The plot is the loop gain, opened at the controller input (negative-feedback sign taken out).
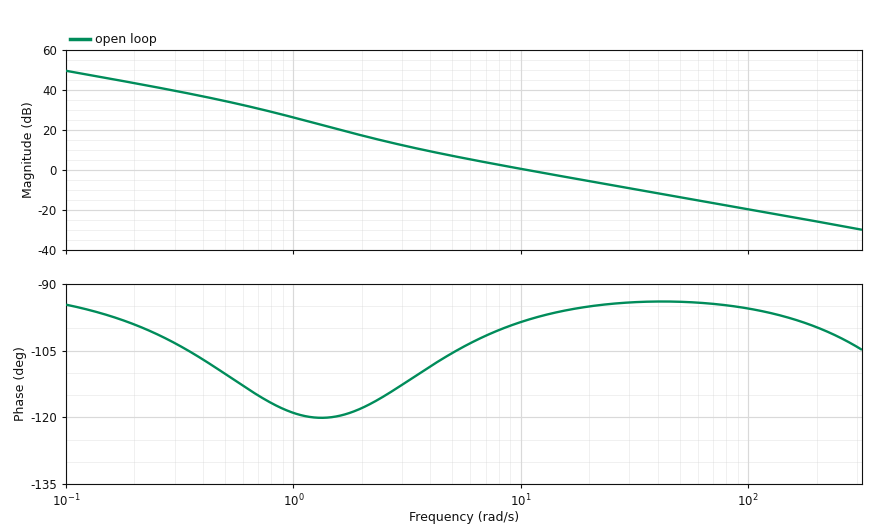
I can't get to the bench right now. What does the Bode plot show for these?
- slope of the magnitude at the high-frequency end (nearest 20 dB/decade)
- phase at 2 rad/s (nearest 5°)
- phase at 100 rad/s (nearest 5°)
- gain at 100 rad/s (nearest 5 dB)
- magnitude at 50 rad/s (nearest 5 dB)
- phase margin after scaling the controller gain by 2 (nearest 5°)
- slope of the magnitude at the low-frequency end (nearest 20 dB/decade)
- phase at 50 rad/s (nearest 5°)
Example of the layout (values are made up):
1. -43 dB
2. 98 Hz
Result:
1. -20 dB/decade
2. -120°
3. -95°
4. -20 dB
5. -15 dB
6. 85°
7. -20 dB/decade
8. -95°
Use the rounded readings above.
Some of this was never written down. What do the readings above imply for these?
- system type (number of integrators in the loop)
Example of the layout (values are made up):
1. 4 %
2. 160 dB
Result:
1. 1
